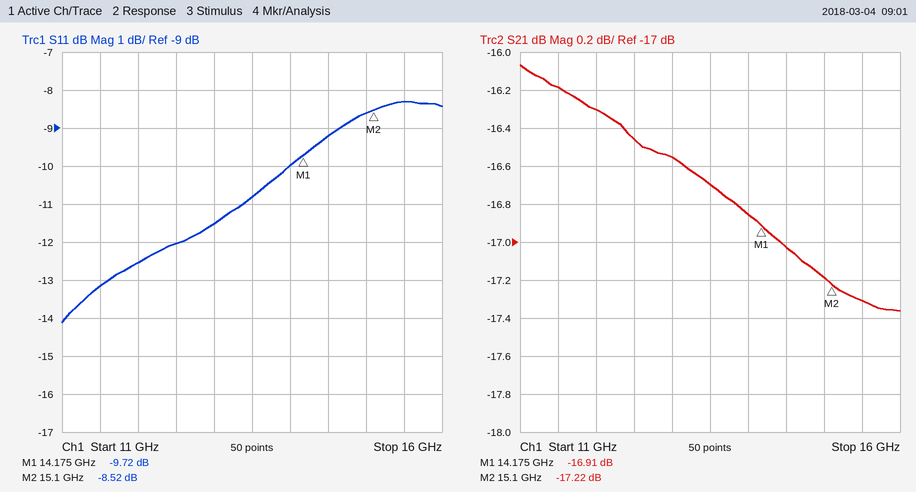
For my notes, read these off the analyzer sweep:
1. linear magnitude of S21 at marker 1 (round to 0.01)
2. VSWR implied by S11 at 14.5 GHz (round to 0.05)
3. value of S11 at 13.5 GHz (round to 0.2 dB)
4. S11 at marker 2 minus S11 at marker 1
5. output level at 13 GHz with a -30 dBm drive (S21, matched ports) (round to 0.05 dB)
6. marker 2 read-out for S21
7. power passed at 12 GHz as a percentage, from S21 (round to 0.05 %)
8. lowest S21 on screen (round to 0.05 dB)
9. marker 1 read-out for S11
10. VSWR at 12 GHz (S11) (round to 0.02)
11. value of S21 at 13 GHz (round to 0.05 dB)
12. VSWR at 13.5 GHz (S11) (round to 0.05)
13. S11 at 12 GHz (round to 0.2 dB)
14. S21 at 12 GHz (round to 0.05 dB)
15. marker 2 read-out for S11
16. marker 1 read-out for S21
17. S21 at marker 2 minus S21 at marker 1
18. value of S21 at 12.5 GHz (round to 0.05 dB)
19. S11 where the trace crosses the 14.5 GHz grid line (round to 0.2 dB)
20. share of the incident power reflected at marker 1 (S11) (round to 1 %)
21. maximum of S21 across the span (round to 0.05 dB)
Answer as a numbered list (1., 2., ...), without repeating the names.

1. 0.14
2. 2.05
3. -10.8 dB
4. 1.20 dB
5. -46.55 dBm
6. -17.22 dB
7. 2.35 %
8. -17.35 dB
9. -9.72 dB
10. 1.62
11. -16.55 dB
12. 1.80
13. -12.6 dB
14. -16.30 dB
15. -8.52 dB
16. -16.91 dB
17. -0.31 dB
18. -16.45 dB
19. -9.2 dB
20. 11 %
21. -16.05 dB
